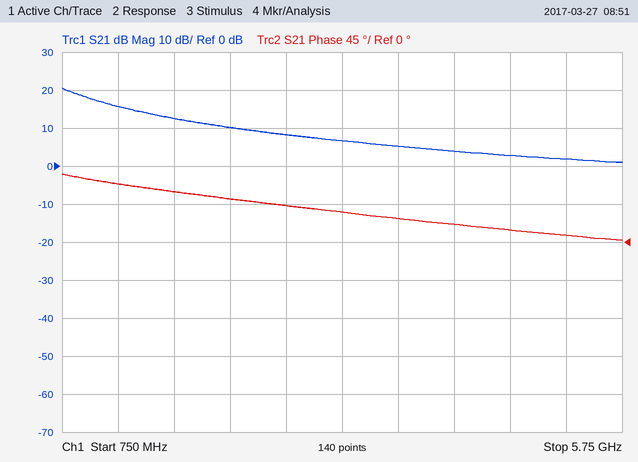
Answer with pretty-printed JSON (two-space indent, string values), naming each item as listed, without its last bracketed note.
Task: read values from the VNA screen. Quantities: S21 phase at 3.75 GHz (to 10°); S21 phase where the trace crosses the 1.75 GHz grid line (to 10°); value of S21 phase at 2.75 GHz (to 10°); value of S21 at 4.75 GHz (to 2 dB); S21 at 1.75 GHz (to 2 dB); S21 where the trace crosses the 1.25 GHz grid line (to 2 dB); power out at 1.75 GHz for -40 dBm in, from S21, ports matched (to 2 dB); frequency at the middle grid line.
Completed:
{
  "S21 phase at 3.75 GHz": "30°",
  "S21 phase where the trace crosses the 1.75 GHz grid line": "60°",
  "value of S21 phase at 2.75 GHz": "40°",
  "value of S21 at 4.75 GHz": "2 dB",
  "S21 at 1.75 GHz": "12 dB",
  "S21 where the trace crosses the 1.25 GHz grid line": "16 dB",
  "power out at 1.75 GHz for -40 dBm in, from S21, ports matched": "-28 dBm",
  "frequency at the middle grid line": "3.25 GHz"
}
